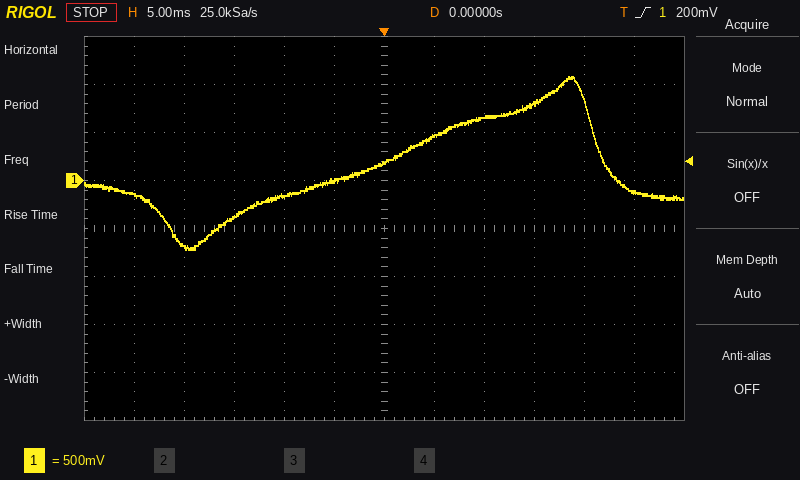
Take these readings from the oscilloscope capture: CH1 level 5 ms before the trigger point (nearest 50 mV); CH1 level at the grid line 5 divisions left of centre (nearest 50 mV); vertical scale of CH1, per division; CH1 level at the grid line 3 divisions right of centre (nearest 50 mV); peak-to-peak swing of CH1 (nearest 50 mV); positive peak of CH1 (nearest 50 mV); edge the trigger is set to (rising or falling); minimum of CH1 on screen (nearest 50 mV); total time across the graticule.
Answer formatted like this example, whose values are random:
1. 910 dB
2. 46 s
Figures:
1. 0 mV
2. -150 mV
3. 500 mV
4. 800 mV
5. 1.80 V
6. 1.10 V
7. rising
8. -700 mV
9. 60 ms
